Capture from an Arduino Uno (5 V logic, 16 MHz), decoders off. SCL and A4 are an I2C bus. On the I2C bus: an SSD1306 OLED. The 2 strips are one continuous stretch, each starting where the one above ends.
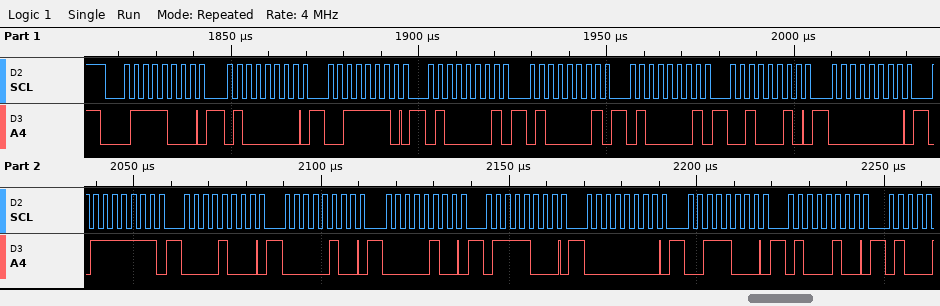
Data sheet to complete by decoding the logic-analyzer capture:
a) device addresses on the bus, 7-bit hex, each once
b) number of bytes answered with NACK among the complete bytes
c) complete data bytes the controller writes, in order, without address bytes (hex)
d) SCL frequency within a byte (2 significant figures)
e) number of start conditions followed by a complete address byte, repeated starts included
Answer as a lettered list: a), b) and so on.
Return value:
a) 0x3C
b) 0
c) 40 3E 41 41 41 22 00 7F 08 04 04 78 00 38 44
d) 400 kHz
e) 1
